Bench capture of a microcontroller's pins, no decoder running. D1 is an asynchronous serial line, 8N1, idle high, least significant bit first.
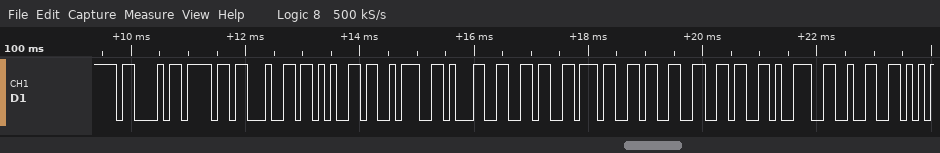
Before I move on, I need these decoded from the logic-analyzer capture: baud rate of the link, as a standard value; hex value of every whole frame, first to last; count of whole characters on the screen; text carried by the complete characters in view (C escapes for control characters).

9600 baud
43 6F 64 65 3A 31 36 37 33 36 39 32
12
"Code:1673692"
